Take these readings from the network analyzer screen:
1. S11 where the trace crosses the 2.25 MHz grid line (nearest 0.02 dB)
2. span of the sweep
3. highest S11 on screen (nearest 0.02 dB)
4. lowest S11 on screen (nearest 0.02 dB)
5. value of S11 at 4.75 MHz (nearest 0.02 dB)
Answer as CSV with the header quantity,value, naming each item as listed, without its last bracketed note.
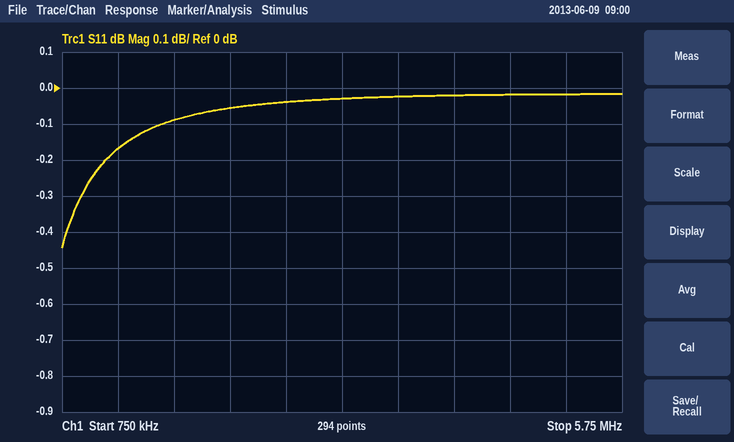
quantity,value
S11 where the trace crosses the 2.25 MHz grid line,-0.06 dB
span of the sweep,5 MHz
highest S11 on screen,-0.02 dB
lowest S11 on screen,-0.44 dB
value of S11 at 4.75 MHz,-0.02 dB
